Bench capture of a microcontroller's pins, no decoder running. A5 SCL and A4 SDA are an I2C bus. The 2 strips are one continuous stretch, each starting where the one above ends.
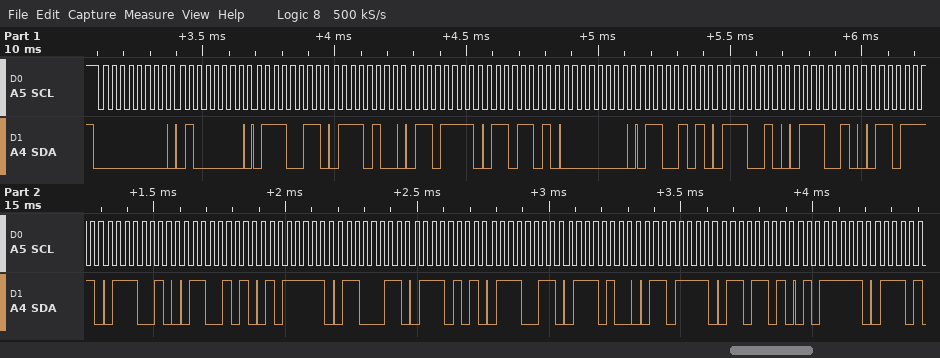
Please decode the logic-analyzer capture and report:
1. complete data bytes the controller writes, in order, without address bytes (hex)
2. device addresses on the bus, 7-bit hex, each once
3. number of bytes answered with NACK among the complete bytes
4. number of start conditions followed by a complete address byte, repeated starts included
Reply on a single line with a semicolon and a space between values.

40 73 74 6F 6D 00 65 72 72 6F 72 65 5F 63 75 73 74 6F 6D 5F; 0x00; 0; 1
